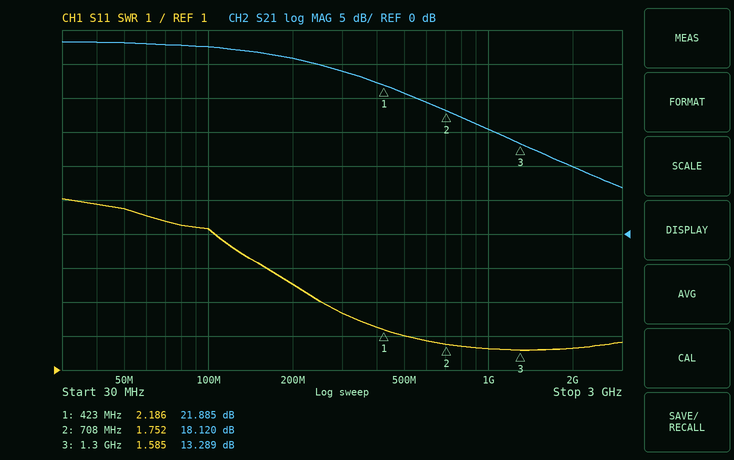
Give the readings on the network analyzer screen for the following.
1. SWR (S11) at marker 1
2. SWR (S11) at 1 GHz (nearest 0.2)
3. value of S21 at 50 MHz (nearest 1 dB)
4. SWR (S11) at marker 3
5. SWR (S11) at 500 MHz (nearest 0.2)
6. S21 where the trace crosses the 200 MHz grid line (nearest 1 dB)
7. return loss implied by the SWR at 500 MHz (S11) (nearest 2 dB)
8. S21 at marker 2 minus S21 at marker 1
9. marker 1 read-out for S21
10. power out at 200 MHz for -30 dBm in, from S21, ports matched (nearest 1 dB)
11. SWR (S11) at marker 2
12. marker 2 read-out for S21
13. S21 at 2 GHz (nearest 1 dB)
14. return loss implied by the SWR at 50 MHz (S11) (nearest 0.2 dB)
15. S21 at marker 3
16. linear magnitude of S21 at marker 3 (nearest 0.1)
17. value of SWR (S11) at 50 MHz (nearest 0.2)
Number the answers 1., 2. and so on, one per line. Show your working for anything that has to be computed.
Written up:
1. 2.186
2. 1.6
3. 28 dB
4. 1.585
5. 2.0
6. 26 dB
7. −20 log10((2 − 1)/(2 + 1)) ≈ 10 dB
8. 18.12 − (21.885) = -3.765 dB
9. 21.885 dB
10. -30 dBm + (26 dB) = -4 dBm
11. 1.752
12. 18.120 dB
13. 10 dB
14. −20 log10((5.8 − 1)/(5.8 + 1)) ≈ 3.0 dB
15. 13.289 dB
16. 10^(13.289/20) ≈ 4.6
17. 5.8
